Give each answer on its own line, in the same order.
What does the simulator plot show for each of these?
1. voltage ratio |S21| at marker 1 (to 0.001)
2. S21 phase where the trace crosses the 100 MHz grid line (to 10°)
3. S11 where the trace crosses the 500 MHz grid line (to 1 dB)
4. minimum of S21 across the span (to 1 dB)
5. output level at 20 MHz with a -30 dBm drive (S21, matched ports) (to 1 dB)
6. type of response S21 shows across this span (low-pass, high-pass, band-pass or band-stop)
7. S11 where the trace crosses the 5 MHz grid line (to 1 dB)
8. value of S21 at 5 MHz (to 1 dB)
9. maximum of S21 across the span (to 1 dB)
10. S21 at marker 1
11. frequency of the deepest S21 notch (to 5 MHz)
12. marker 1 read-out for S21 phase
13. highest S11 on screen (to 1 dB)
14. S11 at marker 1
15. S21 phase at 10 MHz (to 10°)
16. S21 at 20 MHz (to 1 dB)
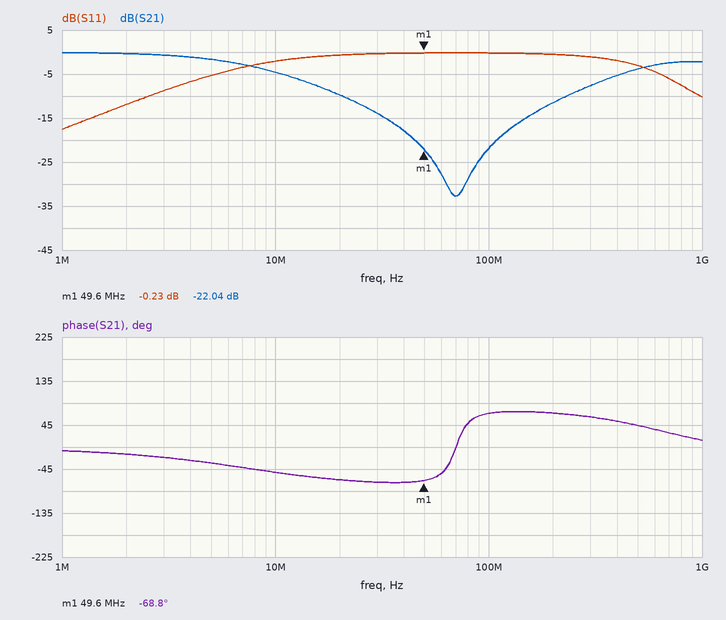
0.079
70°
-3 dB
-33 dB
-40 dBm
band-stop
-5 dB
-2 dB
0 dB
-22.04 dB
70 MHz
-68.8°
0 dB
-0.23 dB
-50°
-10 dB
